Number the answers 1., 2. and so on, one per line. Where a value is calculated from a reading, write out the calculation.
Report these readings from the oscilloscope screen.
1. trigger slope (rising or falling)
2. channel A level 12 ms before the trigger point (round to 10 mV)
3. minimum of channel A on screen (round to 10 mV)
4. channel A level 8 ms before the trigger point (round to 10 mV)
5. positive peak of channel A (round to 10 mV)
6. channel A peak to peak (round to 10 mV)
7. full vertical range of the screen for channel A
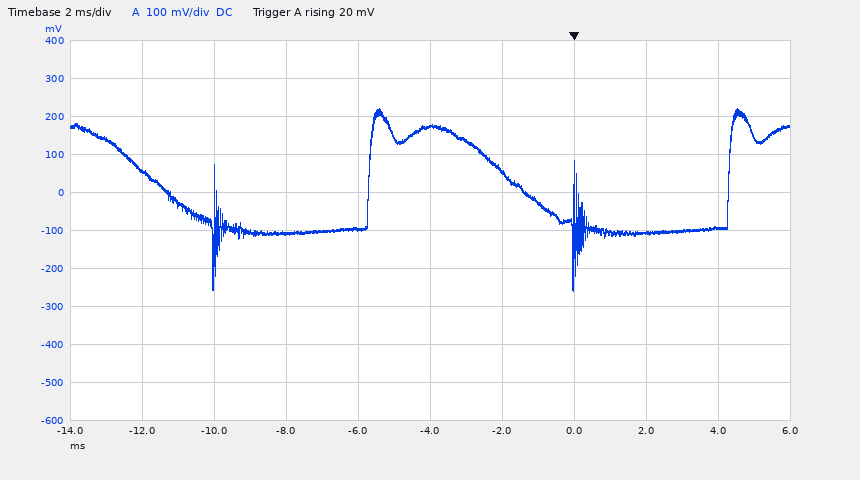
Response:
1. rising
2. 60 mV
3. -260 mV
4. -110 mV
5. 220 mV
6. 220 mV − (-260 mV) = 480 mV
7. 1 V
